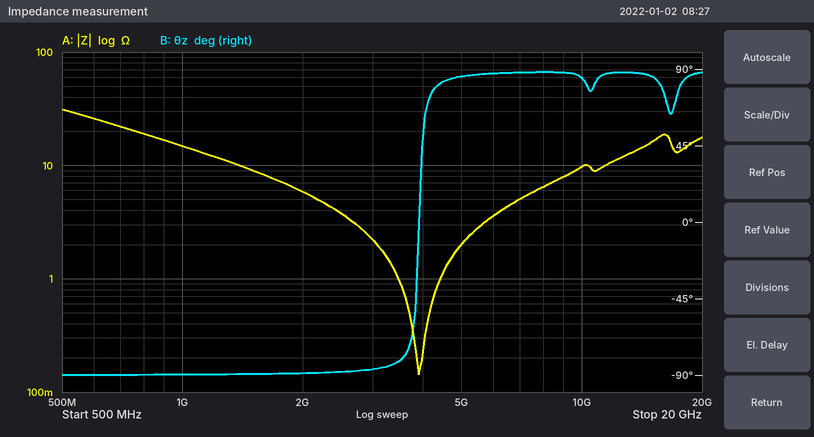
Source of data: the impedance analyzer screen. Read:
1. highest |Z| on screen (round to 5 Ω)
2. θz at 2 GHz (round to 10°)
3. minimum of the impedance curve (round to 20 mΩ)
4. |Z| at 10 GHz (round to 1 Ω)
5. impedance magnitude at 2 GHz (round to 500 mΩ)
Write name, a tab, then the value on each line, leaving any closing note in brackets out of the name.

highest |Z| on screen	30 Ω
θz at 2 GHz	-90°
minimum of the impedance curve	140 mΩ
|Z| at 10 GHz	10 Ω
impedance magnitude at 2 GHz	6.0 Ω
